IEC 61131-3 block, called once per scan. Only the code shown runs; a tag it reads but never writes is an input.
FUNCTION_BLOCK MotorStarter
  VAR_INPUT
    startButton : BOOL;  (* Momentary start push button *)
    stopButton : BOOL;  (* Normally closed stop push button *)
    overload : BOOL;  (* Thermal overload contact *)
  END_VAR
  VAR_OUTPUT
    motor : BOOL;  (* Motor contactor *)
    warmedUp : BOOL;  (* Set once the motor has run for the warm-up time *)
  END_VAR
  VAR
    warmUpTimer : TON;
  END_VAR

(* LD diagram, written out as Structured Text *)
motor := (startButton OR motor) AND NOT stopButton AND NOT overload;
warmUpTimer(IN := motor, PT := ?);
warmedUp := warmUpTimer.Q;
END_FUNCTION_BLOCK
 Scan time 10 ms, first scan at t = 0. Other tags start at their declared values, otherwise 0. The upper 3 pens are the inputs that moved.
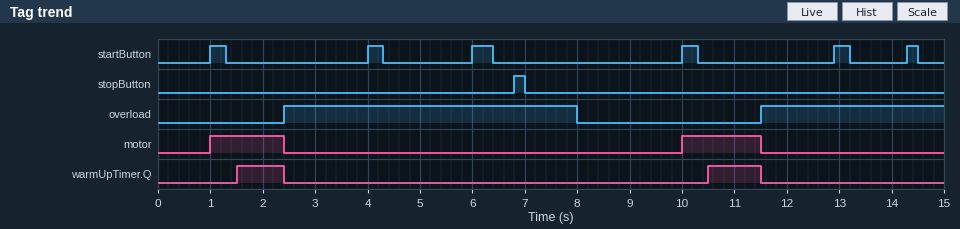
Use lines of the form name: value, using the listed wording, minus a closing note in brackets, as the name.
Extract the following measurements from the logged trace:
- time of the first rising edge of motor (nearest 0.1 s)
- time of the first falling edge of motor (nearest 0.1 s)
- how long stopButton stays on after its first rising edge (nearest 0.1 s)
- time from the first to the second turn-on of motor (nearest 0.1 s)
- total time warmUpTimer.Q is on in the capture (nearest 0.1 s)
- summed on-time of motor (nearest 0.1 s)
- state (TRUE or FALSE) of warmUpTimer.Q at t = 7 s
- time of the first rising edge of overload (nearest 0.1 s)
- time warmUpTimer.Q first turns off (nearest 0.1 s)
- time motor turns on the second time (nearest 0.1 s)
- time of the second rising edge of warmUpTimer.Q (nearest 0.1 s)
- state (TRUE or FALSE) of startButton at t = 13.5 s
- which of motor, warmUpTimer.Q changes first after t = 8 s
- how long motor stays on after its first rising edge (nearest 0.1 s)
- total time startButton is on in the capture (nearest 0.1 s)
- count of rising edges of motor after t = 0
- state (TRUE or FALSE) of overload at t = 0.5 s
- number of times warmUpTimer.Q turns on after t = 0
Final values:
time of the first rising edge of motor: 1.0 s
time of the first falling edge of motor: 2.4 s
how long stopButton stays on after its first rising edge: 0.2 s
time from the first to the second turn-on of motor: 9.0 s
total time warmUpTimer.Q is on in the capture: 1.9 s
summed on-time of motor: 2.9 s
state (TRUE or FALSE) of warmUpTimer.Q at t = 7 s: FALSE
time of the first rising edge of overload: 2.4 s
time warmUpTimer.Q first turns off: 2.4 s
time motor turns on the second time: 10.0 s
time of the second rising edge of warmUpTimer.Q: 10.5 s
state (TRUE or FALSE) of startButton at t = 13.5 s: FALSE
which of motor, warmUpTimer.Q changes first after t = 8 s: motor
how long motor stays on after its first rising edge: 1.4 s
total time startButton is on in the capture: 1.8 s
count of rising edges of motor after t = 0: 2
state (TRUE or FALSE) of overload at t = 0.5 s: FALSE
number of times warmUpTimer.Q turns on after t = 0: 2
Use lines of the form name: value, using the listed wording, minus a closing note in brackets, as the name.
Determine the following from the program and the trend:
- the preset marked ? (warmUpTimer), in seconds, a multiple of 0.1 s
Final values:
the preset marked ? (warmUpTimer), in seconds, a multiple of 0.1 s: 0.5 s
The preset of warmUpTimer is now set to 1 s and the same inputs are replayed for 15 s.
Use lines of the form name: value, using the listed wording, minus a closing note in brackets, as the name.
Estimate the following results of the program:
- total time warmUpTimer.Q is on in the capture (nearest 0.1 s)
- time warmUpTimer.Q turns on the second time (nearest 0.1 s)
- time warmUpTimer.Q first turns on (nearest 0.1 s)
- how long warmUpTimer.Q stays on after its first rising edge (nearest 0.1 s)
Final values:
total time warmUpTimer.Q is on in the capture: 0.9 s
time warmUpTimer.Q turns on the second time: 11.0 s
time warmUpTimer.Q first turns on: 2.0 s
how long warmUpTimer.Q stays on after its first rising edge: 0.4 s
